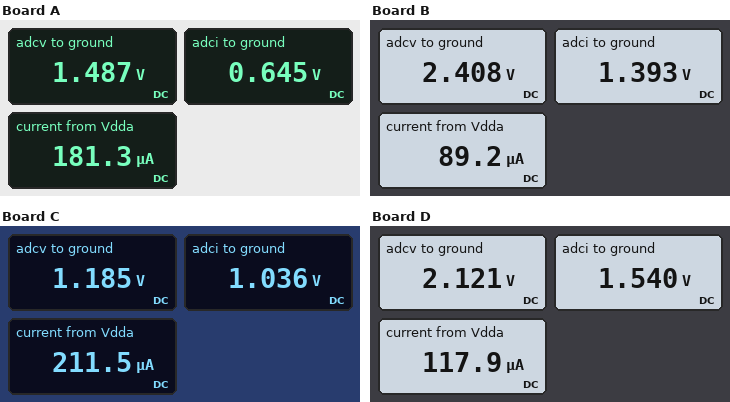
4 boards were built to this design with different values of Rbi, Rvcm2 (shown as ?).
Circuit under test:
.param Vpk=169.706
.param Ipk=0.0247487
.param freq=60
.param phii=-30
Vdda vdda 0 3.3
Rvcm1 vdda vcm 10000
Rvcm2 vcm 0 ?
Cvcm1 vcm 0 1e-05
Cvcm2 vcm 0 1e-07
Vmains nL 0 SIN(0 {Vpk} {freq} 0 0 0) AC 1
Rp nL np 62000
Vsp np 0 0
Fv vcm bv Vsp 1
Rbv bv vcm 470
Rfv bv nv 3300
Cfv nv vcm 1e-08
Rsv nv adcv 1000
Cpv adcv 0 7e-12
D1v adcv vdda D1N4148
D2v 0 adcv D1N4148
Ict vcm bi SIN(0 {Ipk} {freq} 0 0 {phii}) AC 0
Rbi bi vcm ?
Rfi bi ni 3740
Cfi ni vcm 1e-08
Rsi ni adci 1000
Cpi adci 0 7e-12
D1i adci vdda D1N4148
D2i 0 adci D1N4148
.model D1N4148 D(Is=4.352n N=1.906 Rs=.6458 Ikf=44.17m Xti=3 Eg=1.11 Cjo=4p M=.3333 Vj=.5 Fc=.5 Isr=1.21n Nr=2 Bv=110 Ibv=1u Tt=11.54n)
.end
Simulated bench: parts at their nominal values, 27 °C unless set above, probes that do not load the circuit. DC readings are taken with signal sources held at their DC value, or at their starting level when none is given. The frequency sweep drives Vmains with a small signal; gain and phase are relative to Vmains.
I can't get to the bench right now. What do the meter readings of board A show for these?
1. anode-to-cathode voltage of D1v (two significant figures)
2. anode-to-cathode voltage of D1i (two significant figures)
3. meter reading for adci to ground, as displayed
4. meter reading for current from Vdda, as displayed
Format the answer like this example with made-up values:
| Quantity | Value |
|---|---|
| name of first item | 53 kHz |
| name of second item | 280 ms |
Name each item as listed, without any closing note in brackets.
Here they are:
| Quantity | Value |
|---|---|
| anode-to-cathode voltage of D1v | -1.8 V |
| anode-to-cathode voltage of D1i | -2.7 V |
| meter reading for adci to ground, as displayed | 0.645 V |
| meter reading for current from Vdda, as displayed | 181.3 µA |
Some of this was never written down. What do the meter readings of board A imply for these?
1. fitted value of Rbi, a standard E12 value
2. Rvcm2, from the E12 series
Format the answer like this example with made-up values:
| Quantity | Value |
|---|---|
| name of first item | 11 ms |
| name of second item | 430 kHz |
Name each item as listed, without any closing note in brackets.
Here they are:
| Quantity | Value |
|---|---|
| fitted value of Rbi, a standard E12 value | 68 Ω |
| Rvcm2, from the E12 series | 8.2 kΩ |
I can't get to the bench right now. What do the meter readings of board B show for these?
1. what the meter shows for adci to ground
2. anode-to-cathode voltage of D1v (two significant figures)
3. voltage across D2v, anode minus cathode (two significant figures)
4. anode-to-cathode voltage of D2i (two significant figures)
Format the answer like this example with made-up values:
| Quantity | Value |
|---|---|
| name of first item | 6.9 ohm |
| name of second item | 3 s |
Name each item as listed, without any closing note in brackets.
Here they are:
| Quantity | Value |
|---|---|
| what the meter shows for adci to ground | 1.393 V |
| anode-to-cathode voltage of D1v | -890 mV |
| voltage across D2v, anode minus cathode | -2.4 V |
| anode-to-cathode voltage of D2i | -1.4 V |
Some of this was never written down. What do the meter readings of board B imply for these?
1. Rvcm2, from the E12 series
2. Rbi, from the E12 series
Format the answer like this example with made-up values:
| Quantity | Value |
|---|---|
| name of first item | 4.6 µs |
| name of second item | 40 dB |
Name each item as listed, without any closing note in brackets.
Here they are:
| Quantity | Value |
|---|---|
| Rvcm2, from the E12 series | 27 kΩ |
| Rbi, from the E12 series | 82 Ω |
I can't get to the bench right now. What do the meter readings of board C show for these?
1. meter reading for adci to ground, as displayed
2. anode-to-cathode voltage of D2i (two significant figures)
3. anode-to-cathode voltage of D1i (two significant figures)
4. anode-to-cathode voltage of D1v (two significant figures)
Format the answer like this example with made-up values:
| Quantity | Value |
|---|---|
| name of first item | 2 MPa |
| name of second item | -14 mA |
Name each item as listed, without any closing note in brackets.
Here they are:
| Quantity | Value |
|---|---|
| meter reading for adci to ground, as displayed | 1.036 V |
| anode-to-cathode voltage of D2i | -1.0 V |
| anode-to-cathode voltage of D1i | -2.3 V |
| anode-to-cathode voltage of D1v | -2.1 V |
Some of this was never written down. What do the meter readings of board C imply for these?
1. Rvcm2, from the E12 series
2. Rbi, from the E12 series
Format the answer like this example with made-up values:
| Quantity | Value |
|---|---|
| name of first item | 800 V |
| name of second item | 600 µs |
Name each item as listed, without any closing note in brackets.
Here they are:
| Quantity | Value |
|---|---|
| Rvcm2, from the E12 series | 5.6 kΩ |
| Rbi, from the E12 series | 12 Ω |
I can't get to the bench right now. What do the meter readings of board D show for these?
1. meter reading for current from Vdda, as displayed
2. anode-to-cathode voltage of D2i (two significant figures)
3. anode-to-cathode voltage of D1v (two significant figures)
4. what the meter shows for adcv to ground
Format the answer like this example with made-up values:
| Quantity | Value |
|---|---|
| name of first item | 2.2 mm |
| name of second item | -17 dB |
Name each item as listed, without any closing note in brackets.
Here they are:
| Quantity | Value |
|---|---|
| meter reading for current from Vdda, as displayed | 117.9 µA |
| anode-to-cathode voltage of D2i | -1.5 V |
| anode-to-cathode voltage of D1v | -1.2 V |
| what the meter shows for adcv to ground | 2.121 V |
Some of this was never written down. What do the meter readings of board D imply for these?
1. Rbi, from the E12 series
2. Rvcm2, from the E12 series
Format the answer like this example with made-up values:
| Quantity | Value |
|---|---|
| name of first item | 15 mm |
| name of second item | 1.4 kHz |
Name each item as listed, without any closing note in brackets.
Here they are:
| Quantity | Value |
|---|---|
| Rbi, from the E12 series | 47 Ω |
| Rvcm2, from the E12 series | 18 kΩ |
